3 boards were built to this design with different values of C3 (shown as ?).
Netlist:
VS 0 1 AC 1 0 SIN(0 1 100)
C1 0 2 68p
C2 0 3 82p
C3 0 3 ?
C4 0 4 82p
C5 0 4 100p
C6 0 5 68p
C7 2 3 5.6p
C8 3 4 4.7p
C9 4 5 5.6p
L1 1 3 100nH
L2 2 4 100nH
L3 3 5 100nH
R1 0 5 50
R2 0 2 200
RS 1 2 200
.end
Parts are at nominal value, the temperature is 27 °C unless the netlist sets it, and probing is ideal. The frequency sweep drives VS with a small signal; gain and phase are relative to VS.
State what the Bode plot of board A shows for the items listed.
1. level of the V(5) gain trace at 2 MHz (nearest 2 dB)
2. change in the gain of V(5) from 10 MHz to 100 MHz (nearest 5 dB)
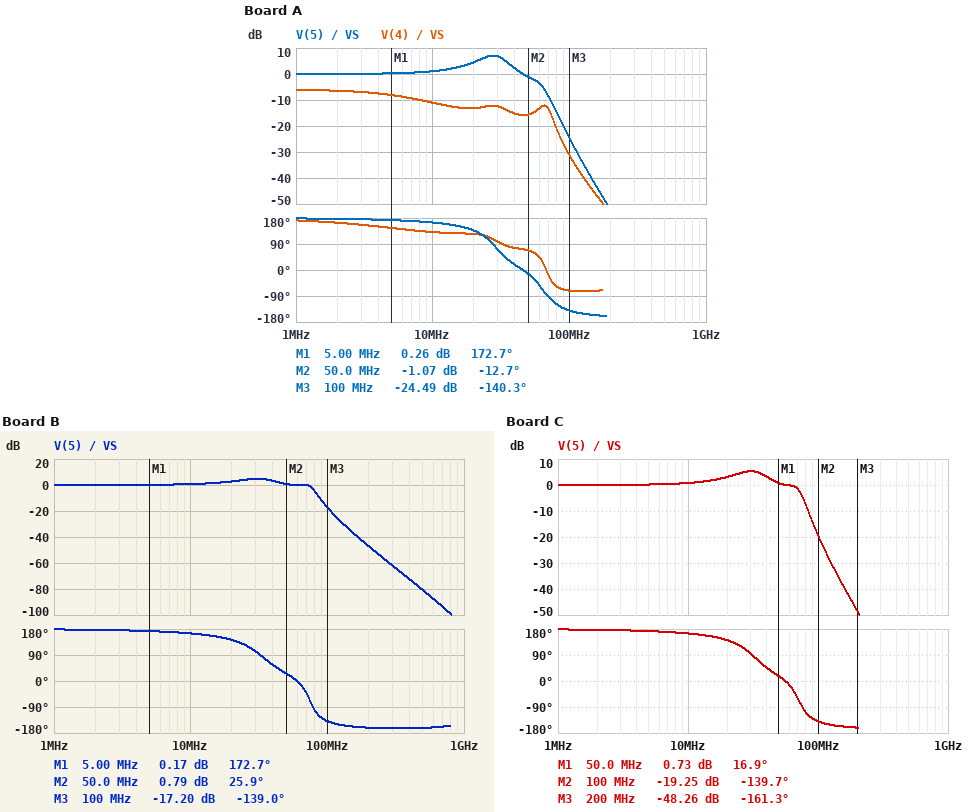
0 dB
-25 dB
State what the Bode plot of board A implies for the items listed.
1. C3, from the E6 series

150 pF
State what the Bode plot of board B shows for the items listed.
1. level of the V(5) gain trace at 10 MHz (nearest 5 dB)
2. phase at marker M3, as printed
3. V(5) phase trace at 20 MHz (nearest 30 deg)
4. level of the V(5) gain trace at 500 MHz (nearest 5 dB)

0 dB
-139.0 deg
150 deg
-80 dB
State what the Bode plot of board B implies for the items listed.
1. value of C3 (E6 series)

47 pF
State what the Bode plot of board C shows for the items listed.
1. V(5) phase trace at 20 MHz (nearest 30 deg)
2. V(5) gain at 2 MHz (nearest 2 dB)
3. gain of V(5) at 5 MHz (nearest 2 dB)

150 deg
0 dB
0 dB
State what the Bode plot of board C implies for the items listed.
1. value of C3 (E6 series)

68 pF
